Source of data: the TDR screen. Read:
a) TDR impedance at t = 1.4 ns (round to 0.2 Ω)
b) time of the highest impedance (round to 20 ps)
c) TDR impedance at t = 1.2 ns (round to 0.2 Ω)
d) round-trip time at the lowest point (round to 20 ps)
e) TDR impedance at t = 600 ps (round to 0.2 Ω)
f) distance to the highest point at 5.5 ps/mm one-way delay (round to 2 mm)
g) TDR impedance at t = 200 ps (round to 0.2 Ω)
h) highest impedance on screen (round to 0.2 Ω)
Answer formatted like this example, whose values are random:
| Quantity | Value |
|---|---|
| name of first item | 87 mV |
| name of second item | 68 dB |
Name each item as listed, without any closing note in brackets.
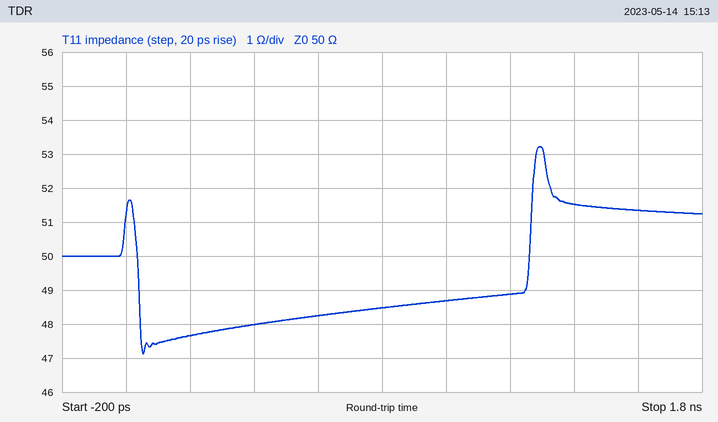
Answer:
| Quantity | Value |
|---|---|
| TDR impedance at t = 1.4 ns | 51.6 Ω |
| time of the highest impedance | 1.30 ns |
| TDR impedance at t = 1.2 ns | 48.8 Ω |
| round-trip time at the lowest point | 60 ps |
| TDR impedance at t = 600 ps | 48.2 Ω |
| distance to the highest point at 5.5 ps/mm one-way delay | 118 mm |
| TDR impedance at t = 200 ps | 47.6 Ω |
| highest impedance on screen | 53.2 Ω |
